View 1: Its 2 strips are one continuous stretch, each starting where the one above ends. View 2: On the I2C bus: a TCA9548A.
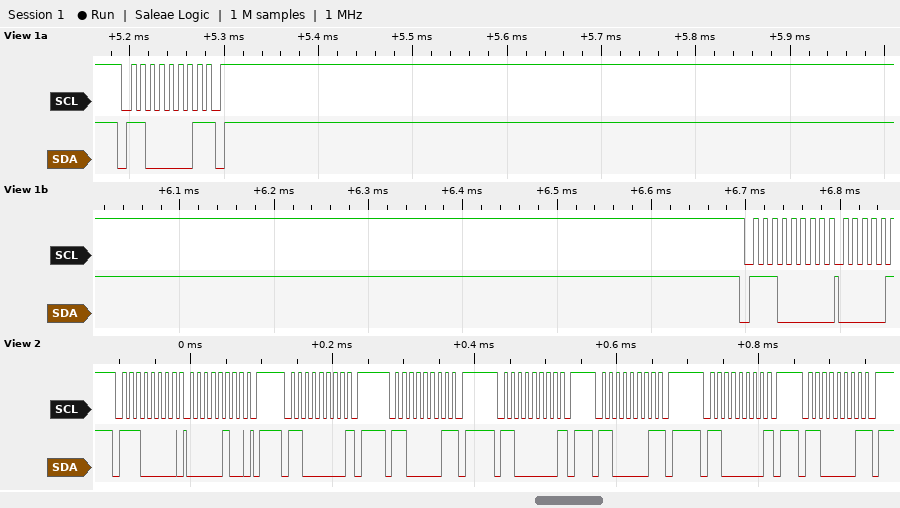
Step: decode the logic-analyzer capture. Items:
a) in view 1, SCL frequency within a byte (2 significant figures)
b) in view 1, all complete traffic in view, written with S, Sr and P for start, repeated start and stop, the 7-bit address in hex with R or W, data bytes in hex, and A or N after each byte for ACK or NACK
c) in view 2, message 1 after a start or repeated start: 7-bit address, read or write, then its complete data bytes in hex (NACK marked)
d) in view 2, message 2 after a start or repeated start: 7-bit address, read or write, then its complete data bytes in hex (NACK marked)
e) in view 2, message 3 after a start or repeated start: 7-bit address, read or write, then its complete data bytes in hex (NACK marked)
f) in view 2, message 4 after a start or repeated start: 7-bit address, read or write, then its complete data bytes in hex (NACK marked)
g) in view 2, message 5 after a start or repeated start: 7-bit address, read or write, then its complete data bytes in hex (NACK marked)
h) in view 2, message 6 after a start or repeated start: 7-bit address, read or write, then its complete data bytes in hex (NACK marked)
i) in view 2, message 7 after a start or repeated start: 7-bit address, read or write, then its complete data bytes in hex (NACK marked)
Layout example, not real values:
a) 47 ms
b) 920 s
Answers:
a) 100 kHz
b) S 60R N P S 70W A
c) 0x70 write: 04
d) 0x60 write NACK
e) 0x60 read NACK
f) 0x60 write NACK
g) 0x60 read NACK
h) 0x60 write NACK
i) 0x60 read NACK
